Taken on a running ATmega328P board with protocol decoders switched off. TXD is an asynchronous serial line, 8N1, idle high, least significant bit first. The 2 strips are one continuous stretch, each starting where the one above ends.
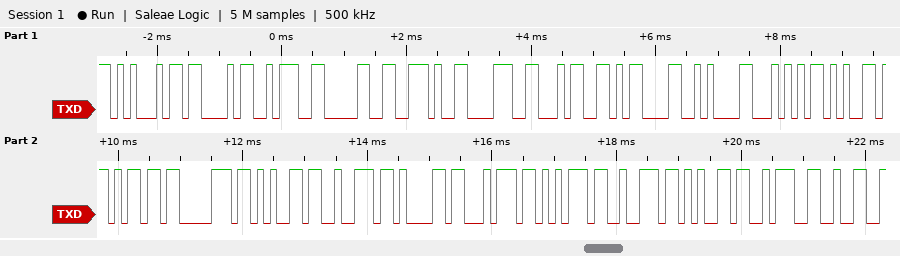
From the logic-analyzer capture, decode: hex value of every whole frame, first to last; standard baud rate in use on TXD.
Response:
45 43 3A 30 2E 38 34 0D 0A 54 65 6D 70 65 72 61 74 75 72 65 3A 32
9600 baud
